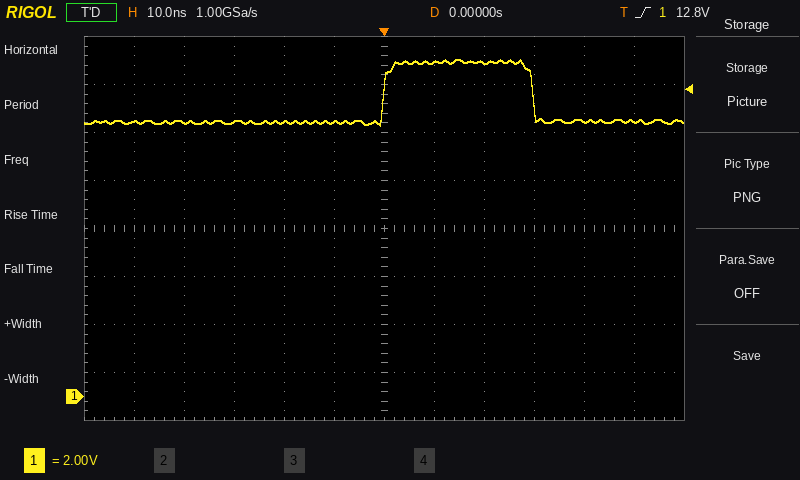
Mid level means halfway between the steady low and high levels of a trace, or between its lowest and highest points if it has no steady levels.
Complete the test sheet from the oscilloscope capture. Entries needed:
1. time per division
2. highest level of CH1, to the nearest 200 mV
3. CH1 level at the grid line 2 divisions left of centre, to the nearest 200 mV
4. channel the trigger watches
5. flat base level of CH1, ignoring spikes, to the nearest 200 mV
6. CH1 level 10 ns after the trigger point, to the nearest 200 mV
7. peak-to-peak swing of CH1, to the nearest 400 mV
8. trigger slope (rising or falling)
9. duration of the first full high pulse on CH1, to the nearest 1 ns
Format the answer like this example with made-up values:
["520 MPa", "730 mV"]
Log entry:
["10 ns", "14.0 V", "11.4 V", "CH1", "11.4 V", "14.0 V", "2.8 V", "rising", "30 ns"]
